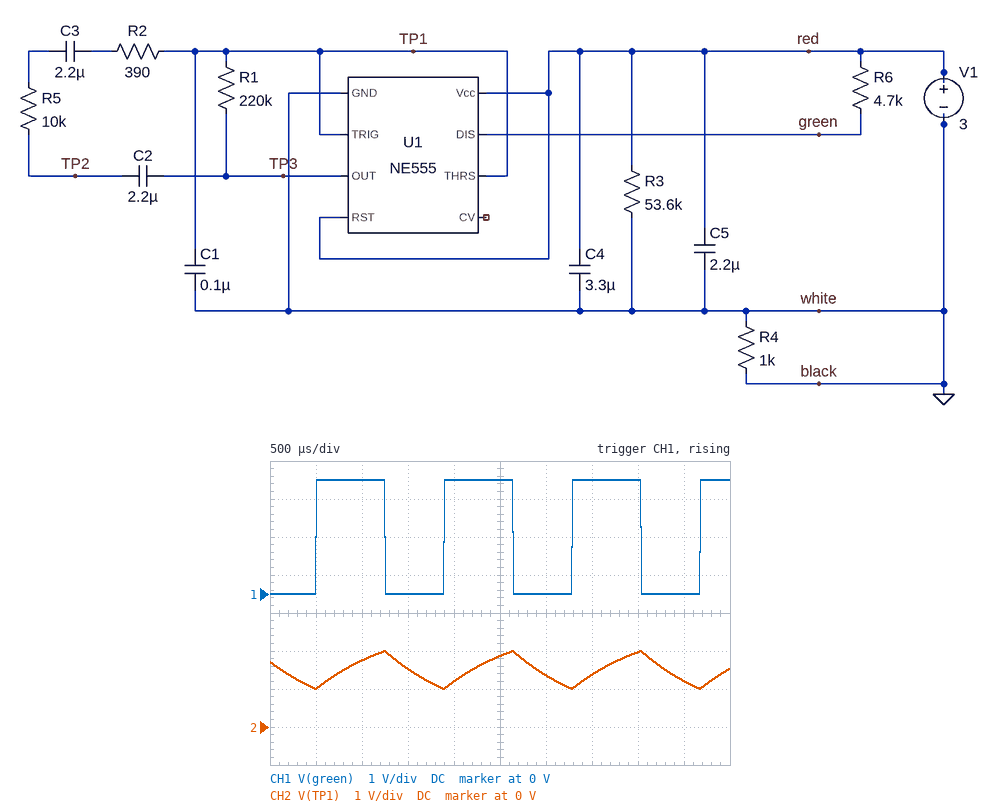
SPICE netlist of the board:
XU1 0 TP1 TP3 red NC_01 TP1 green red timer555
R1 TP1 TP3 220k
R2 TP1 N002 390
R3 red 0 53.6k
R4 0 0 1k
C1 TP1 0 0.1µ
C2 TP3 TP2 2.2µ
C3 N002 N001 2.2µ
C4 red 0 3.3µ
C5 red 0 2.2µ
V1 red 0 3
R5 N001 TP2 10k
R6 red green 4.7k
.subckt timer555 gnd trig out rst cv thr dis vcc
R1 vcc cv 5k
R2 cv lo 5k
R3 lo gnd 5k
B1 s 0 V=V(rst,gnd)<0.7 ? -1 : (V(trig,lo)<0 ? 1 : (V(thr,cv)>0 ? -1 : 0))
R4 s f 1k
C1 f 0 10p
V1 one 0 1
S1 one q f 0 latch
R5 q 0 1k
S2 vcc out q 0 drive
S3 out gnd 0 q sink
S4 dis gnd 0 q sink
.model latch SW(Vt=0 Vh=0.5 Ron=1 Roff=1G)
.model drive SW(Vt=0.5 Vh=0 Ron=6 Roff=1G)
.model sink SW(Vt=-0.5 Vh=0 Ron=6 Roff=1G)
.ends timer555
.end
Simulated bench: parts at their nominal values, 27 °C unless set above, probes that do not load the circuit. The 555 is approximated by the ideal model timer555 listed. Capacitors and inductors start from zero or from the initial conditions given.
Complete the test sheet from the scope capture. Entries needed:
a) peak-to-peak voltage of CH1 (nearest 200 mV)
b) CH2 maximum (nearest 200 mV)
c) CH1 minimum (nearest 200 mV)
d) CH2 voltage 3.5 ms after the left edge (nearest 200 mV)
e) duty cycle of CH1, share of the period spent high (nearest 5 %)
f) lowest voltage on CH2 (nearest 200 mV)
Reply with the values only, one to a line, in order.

3.0 V
2.0 V
0 V
1.4 V
55 %
1.0 V
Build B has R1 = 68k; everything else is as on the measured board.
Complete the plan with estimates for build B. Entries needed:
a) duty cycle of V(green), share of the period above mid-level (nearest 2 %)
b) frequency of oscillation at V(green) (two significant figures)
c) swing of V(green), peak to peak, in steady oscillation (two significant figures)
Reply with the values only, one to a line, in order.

52 %
790 Hz
3.0 V
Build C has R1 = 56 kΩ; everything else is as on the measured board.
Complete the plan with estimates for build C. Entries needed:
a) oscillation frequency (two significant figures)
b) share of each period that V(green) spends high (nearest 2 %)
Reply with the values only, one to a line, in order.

820 Hz
52 %
